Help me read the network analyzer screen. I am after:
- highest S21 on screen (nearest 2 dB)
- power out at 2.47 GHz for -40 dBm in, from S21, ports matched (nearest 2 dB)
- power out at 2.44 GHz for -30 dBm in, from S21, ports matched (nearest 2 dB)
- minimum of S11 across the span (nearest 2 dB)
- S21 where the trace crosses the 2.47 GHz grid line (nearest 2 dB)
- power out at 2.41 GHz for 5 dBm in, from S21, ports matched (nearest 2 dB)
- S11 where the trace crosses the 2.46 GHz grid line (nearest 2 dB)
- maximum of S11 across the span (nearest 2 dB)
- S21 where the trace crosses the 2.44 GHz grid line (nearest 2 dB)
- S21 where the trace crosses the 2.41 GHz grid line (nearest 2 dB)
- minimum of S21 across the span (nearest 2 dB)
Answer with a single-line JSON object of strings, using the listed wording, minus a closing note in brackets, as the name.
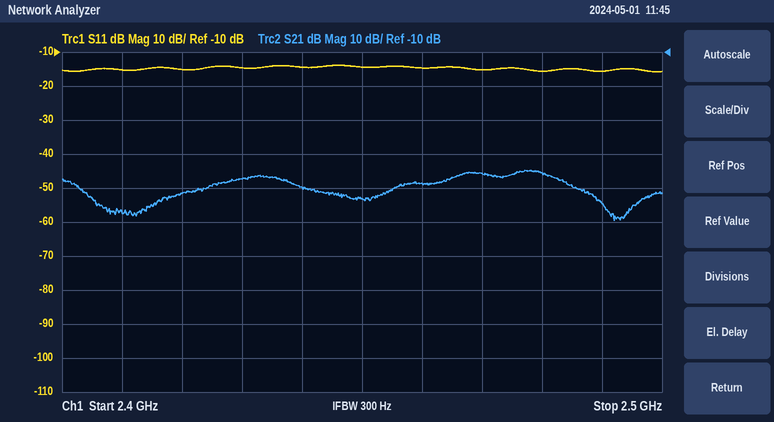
{"highest S21 on screen": "-44 dB", "power out at 2.47 GHz for -40 dBm in, from S21, ports matched": "-86 dBm", "power out at 2.44 GHz for -30 dBm in, from S21, ports matched": "-80 dBm", "minimum of S11 across the span": "-16 dB", "S21 where the trace crosses the 2.47 GHz grid line": "-46 dB", "power out at 2.41 GHz for 5 dBm in, from S21, ports matched": "-52 dBm", "S11 where the trace crosses the 2.46 GHz grid line": "-14 dB", "maximum of S11 across the span": "-14 dB", "S21 where the trace crosses the 2.44 GHz grid line": "-50 dB", "S21 where the trace crosses the 2.41 GHz grid line": "-58 dB", "minimum of S21 across the span": "-60 dB"}
